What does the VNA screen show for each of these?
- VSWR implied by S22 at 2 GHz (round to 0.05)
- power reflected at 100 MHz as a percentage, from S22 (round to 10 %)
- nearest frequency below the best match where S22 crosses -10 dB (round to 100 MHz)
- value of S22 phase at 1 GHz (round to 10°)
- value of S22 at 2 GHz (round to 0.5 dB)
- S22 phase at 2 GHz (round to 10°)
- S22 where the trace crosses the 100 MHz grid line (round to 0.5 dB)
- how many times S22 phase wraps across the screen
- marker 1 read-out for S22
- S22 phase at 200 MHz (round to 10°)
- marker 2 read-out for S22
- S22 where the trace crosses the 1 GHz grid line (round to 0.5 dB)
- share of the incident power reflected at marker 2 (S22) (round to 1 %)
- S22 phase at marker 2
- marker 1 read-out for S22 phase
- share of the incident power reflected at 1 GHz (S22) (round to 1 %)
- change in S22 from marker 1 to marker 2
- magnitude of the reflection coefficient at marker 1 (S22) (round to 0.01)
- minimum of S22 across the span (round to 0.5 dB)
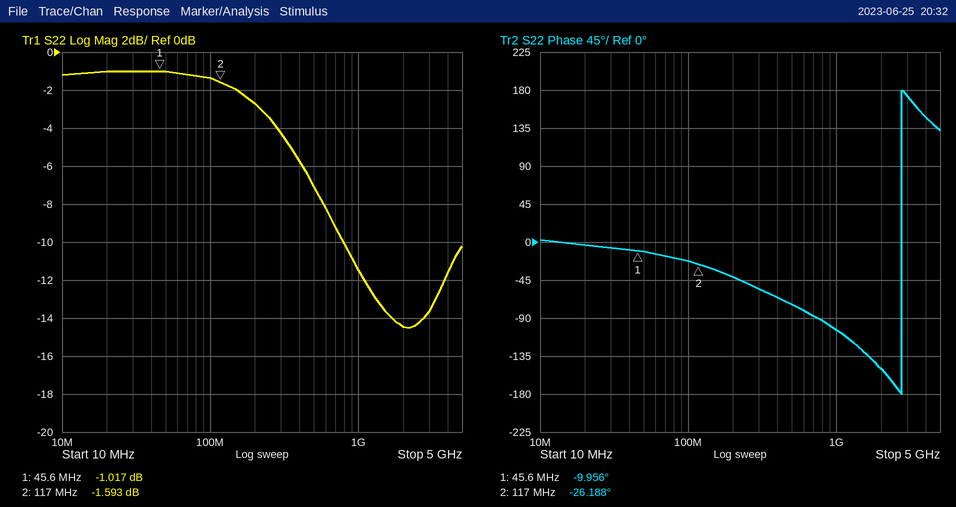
1.45
70 %
800 MHz
-100°
-14.5 dB
-150°
-1.5 dB
1
-1.017 dB
-40°
-1.593 dB
-11.5 dB
69 %
-26.188°
-9.956°
7 %
-0.576 dB
0.89
-14.5 dB
